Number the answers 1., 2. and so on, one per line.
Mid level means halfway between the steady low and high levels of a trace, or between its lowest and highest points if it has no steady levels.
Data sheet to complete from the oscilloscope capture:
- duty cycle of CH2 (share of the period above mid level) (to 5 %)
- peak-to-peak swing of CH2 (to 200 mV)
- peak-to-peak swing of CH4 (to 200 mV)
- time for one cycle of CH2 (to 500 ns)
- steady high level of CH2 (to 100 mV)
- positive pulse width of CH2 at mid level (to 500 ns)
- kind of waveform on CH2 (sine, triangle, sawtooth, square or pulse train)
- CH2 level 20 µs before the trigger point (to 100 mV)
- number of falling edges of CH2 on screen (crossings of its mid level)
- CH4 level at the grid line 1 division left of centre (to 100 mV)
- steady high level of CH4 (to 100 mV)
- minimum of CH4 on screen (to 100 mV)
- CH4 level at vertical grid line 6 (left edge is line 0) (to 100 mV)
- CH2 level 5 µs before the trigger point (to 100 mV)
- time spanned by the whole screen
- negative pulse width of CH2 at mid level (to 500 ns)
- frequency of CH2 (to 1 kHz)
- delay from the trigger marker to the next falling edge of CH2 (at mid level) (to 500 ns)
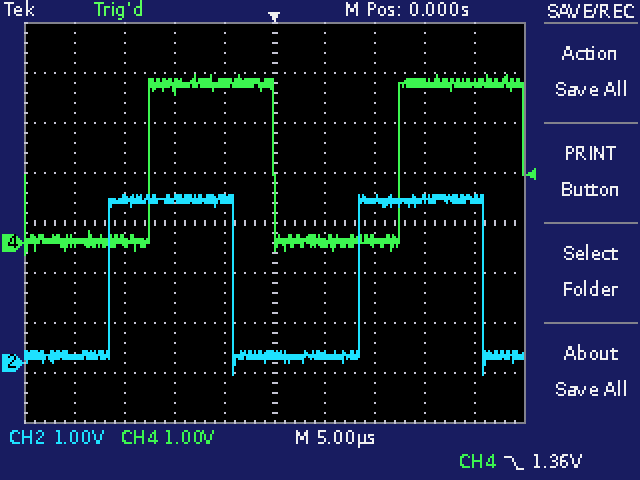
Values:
1. 50 %
2. 3.6 V
3. 3.6 V
4. 25.0 µs
5. 3.3 V
6. 12.5 µs
7. square
8. 100 mV
9. 2
10. 3.2 V
11. 3.2 V
12. -200 mV
13. 0.0 V
14. 3.3 V
15. 50 µs
16. 12.5 µs
17. 40 kHz
18. 21.0 µs
